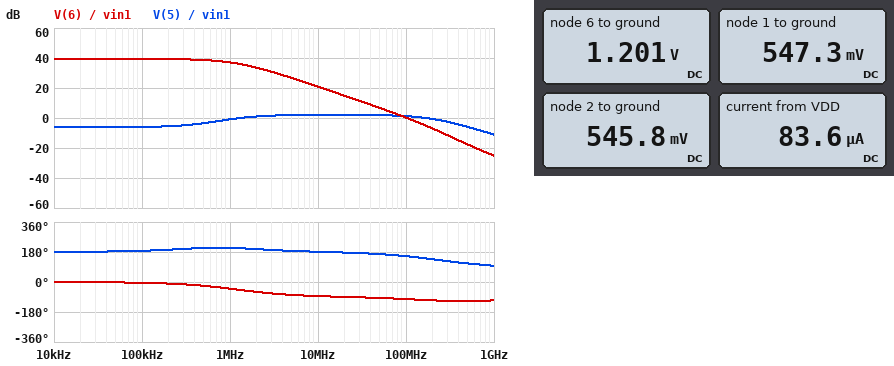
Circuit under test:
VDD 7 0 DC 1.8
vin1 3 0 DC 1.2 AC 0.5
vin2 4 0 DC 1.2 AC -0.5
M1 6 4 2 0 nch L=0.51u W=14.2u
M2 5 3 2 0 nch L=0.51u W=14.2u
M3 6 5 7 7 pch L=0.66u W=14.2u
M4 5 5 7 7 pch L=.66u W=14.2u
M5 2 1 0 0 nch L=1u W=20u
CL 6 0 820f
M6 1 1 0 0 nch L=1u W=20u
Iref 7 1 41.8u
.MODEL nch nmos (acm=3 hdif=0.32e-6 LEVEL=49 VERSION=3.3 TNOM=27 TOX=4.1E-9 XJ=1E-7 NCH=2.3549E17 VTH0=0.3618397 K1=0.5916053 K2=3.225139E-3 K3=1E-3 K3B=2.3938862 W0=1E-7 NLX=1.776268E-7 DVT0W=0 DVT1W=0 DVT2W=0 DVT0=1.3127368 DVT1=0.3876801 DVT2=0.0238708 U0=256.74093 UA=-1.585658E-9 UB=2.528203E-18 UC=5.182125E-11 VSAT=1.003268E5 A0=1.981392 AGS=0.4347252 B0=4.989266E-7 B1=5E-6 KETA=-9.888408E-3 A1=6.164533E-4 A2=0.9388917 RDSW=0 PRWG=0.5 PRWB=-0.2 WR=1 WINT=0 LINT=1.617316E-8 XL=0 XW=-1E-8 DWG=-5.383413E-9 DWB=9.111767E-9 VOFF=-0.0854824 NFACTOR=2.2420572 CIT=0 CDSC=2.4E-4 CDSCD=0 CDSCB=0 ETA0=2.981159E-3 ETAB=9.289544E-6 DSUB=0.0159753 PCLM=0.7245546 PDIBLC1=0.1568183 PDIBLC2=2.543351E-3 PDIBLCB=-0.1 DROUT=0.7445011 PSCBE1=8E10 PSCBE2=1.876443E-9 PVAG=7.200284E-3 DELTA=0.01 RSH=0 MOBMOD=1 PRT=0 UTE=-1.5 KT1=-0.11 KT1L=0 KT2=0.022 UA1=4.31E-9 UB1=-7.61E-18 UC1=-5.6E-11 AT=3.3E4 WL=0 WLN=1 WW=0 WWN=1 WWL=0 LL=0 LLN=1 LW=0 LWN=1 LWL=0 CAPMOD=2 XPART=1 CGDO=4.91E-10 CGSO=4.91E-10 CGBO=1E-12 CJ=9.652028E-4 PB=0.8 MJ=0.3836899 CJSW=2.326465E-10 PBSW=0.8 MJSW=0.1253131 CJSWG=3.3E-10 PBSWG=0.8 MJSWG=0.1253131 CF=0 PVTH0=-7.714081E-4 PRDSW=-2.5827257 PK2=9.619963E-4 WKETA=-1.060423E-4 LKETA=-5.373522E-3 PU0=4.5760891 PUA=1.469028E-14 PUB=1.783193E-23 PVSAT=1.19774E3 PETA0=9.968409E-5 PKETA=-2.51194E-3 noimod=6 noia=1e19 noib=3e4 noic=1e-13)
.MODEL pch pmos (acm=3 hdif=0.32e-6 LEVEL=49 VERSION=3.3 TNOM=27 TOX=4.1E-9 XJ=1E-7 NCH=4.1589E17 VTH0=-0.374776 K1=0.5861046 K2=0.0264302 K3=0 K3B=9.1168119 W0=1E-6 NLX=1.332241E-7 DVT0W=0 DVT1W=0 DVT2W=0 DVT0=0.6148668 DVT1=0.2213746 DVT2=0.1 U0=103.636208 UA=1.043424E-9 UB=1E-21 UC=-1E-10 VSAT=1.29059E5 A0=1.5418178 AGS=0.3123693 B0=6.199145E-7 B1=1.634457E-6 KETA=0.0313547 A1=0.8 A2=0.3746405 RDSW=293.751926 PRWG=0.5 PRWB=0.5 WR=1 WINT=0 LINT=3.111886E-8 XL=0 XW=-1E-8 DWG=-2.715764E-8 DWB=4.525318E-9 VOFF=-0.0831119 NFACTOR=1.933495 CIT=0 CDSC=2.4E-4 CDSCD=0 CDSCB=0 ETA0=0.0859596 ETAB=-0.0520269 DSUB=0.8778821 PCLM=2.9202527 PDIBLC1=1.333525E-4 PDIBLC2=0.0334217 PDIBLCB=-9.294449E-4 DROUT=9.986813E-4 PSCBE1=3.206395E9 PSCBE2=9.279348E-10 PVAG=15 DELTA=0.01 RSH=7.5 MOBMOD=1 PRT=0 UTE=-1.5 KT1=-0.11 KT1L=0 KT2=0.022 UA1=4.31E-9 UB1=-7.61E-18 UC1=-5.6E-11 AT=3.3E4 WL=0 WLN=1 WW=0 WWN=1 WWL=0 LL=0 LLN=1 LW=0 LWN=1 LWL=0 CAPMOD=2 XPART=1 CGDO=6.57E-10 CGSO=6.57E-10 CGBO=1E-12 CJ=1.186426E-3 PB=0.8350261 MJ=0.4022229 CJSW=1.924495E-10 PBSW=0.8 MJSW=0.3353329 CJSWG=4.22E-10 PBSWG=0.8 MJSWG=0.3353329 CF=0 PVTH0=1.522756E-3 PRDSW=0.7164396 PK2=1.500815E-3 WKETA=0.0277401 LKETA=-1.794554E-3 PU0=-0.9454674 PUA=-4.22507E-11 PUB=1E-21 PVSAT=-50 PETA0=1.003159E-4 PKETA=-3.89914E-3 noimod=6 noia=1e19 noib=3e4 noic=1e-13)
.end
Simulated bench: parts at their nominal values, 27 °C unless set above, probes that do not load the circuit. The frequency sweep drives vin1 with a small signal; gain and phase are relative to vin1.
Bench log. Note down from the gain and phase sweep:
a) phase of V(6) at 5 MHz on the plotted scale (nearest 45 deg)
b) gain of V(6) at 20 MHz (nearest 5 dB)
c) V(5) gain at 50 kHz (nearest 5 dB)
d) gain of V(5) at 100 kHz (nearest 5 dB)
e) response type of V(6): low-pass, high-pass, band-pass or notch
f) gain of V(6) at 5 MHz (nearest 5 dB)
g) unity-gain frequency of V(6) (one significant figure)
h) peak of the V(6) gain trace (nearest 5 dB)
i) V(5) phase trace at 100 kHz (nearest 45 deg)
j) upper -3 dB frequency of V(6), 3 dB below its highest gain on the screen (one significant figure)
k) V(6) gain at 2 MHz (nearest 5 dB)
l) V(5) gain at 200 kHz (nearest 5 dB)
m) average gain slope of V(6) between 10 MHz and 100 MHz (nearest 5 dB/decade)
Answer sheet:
-90 deg
15 dB
-5 dB
-5 dB
low-pass
25 dB
100 MHz
40 dB
180 deg
1 MHz
35 dB
-5 dB
-20 dB/decade
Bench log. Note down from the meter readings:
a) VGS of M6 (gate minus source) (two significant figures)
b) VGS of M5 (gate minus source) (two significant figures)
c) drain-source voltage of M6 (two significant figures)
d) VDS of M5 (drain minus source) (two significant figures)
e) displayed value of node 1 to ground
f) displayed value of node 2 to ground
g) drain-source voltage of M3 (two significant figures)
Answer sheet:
550 mV
550 mV
550 mV
550 mV
547.3 mV
545.8 mV
-600 mV
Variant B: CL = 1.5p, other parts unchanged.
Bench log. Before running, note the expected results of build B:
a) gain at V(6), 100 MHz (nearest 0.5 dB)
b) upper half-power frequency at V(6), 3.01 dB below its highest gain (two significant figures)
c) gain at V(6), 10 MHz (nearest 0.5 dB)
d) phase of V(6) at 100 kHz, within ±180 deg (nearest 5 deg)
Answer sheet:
-4.5 dB
670 kHz
16.0 dB
-10 deg
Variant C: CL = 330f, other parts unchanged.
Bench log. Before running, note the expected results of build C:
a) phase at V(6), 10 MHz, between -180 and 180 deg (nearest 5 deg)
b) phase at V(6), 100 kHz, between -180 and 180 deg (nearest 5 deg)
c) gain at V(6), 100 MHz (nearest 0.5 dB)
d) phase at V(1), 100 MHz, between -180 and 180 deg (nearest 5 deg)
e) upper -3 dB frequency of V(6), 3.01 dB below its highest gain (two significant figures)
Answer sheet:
-75 deg
0 deg
7.5 dB
65 deg
2.7 MHz
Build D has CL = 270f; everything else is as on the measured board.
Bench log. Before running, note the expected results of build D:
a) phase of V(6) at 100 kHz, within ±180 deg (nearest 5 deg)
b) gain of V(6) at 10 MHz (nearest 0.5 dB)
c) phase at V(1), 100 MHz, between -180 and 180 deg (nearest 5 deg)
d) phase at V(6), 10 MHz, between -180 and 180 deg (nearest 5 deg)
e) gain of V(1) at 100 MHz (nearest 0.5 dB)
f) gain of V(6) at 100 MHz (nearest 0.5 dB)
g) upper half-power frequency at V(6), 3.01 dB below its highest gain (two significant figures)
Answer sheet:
0 deg
29.0 dB
65 deg
-75 deg
-55.0 dB
9.0 dB
3.2 MHz
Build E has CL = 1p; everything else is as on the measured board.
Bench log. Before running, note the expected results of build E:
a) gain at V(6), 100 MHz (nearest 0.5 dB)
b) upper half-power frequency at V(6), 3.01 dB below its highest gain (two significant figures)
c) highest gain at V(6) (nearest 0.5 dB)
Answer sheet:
-1.5 dB
990 kHz
39.5 dB
